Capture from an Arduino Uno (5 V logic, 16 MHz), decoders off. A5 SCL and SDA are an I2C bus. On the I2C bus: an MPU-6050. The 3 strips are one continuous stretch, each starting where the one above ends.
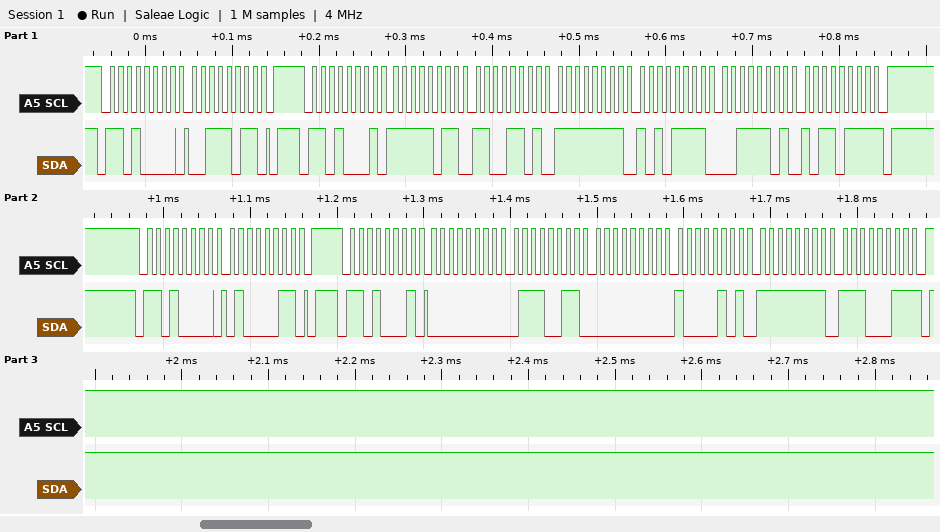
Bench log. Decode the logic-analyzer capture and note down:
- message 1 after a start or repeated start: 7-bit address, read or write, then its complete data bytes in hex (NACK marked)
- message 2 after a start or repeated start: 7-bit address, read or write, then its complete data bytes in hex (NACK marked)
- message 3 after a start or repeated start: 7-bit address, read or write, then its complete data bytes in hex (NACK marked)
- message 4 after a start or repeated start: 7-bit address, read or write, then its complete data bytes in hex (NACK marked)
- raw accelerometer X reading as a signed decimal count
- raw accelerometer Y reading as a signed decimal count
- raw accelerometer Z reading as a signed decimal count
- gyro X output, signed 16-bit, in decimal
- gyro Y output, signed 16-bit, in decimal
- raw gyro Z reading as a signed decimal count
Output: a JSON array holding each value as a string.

["0x68 write: 3B", "0x68 read: FB CD FF AF 3D B7 NACK", "0x68 write: 43", "0x68 read: 00 73 00 85 FF E3 NACK", "-1075", "-81", "15799", "115", "133", "-29"]
